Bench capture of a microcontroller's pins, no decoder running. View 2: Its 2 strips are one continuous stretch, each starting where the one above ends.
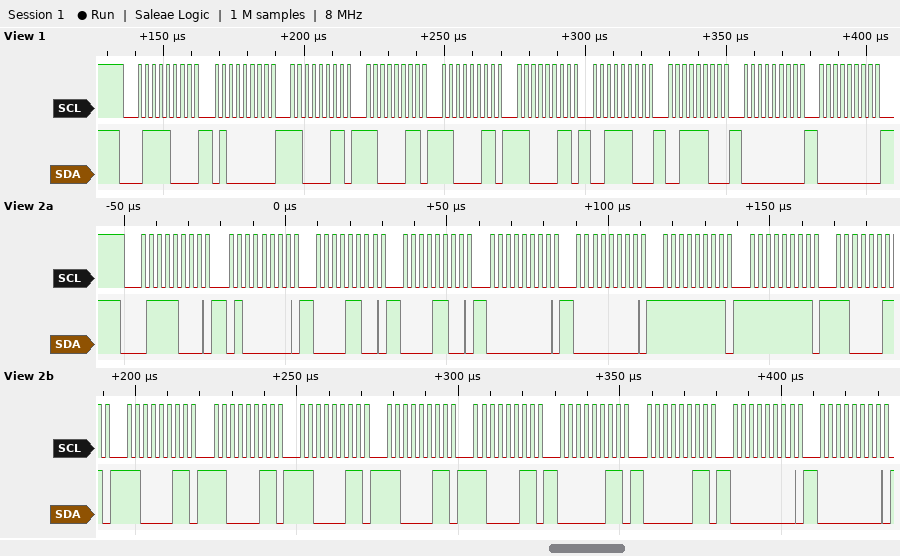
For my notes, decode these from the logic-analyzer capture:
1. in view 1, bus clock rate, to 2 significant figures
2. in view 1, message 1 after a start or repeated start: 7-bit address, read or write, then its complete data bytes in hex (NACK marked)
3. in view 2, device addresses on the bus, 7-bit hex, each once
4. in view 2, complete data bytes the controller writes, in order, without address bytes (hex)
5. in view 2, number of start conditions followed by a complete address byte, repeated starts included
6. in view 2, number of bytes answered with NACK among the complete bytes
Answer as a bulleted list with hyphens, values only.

- 400 kHz
- 0x3C write: 40 C3 C3 C3 C3 3C 3C 00 00
- 0x3C
- 40 0C 0C 00 00 FF FF C3 C3 C3 C3 C3 C3 03 03 00 00
- 1
- 0
